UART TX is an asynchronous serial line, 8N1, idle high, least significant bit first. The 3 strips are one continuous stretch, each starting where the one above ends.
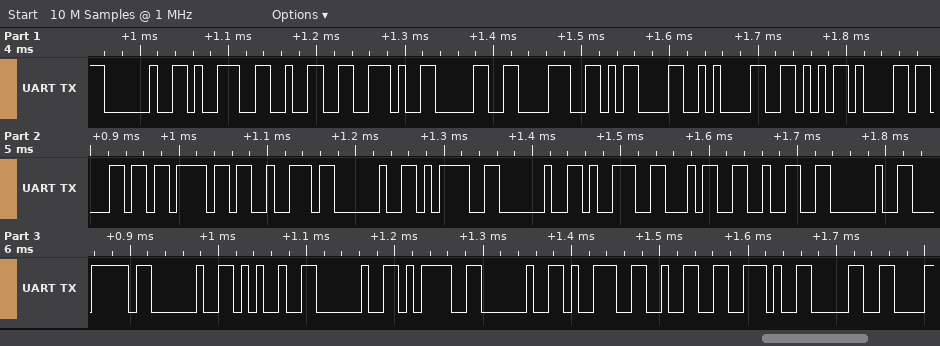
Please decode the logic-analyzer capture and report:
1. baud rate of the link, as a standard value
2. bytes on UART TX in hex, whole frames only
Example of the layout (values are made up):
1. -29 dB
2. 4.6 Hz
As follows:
1. 115200 baud
2. 20 39 32 2E 30 38 0D 0A 56 61 6C 6F 72 20 3D 20 39 34 32 20 7C 20 25 20 3D 20 39 32 2E 30
